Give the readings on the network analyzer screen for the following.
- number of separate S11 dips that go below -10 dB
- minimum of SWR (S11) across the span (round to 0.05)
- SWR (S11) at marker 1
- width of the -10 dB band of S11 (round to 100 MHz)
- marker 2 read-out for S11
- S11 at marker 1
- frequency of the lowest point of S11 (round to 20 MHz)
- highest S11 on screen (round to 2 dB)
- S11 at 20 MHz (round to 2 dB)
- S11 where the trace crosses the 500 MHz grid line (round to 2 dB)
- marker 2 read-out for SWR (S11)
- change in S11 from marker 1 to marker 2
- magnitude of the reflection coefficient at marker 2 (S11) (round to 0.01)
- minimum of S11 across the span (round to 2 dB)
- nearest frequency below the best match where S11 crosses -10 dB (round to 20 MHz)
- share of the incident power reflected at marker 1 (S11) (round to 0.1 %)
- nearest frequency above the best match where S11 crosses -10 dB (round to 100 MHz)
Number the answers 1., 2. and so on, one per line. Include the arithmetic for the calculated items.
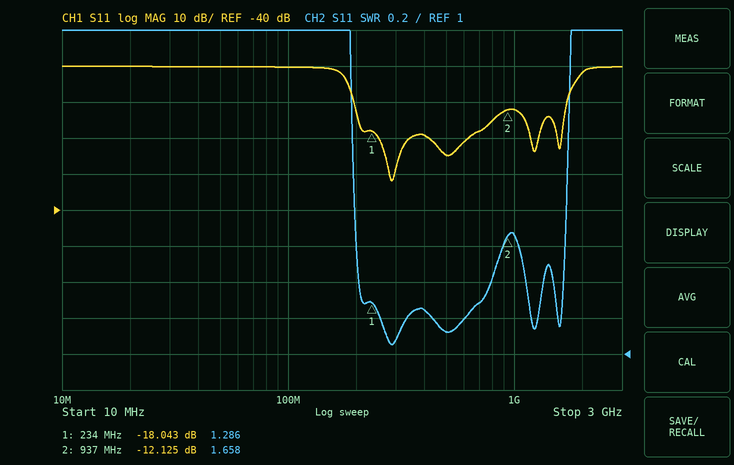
1. 4
2. 1.05
3. 1.286
4. 1.7 GHz − 200 MHz = 1.50 GHz
5. -12.125 dB
6. -18.043 dB
7. 280 MHz
8. 0 dB
9. 0 dB
10. -24 dB
11. 1.658
12. -12.125 − (-18.043) = 5.918 dB
13. 10^(-12.125/20) ≈ 0.25
14. -32 dB
15. 200 MHz
16. 10^(-18.043/10) ≈ 1.6 %
17. 1.7 GHz
